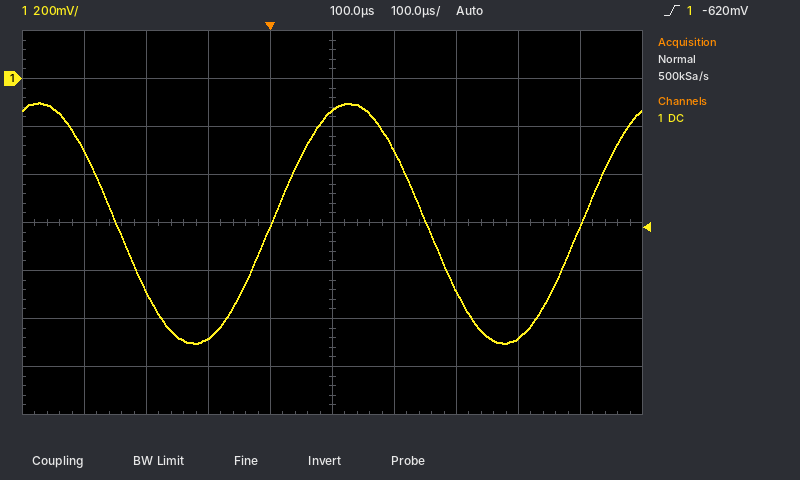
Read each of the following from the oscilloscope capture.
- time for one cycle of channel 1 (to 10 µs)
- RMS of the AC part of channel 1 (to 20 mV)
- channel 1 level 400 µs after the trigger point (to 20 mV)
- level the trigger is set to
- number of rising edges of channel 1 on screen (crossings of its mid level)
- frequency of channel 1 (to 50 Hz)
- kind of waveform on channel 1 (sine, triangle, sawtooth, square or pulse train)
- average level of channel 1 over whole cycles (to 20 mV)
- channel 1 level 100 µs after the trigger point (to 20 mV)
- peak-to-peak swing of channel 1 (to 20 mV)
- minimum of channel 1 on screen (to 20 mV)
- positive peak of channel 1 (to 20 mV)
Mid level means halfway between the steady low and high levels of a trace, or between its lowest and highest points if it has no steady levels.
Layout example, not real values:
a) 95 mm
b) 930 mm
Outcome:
a) 500 µs
b) 360 mV
c) -1.08 V
d) -620 mV
e) 2
f) 2.00 kHz
g) sine
h) -600 mV
i) -140 mV
j) 1.00 V
k) -1.10 V
l) -100 mV
